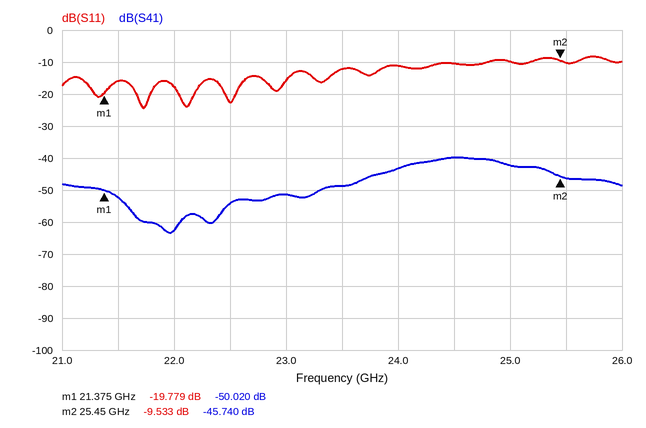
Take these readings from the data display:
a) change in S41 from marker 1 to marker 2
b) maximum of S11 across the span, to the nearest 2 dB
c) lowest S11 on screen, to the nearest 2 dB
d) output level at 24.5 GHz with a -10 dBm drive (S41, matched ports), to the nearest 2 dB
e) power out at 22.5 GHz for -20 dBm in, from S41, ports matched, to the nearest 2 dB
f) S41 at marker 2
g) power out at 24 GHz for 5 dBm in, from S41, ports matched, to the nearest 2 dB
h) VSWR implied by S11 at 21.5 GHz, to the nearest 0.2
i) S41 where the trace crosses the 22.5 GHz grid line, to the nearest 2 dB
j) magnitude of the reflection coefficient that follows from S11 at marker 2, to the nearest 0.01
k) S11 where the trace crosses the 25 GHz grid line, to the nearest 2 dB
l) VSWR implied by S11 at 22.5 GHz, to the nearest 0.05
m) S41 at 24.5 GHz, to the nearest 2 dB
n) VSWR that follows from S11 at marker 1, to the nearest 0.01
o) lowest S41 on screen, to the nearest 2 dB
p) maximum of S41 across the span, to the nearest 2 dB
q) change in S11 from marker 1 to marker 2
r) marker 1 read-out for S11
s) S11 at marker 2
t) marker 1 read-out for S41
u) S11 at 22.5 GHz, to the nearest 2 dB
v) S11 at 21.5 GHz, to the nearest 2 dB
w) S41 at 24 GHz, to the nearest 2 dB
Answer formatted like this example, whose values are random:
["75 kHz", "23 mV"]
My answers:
["4.280 dB", "-8 dB", "-24 dB", "-50 dBm", "-74 dBm", "-45.740 dB", "-38 dBm", "1.4", "-54 dB", "0.33", "-10 dB", "1.15", "-40 dB", "1.23", "-64 dB", "-40 dB", "10.246 dB", "-19.779 dB", "-9.533 dB", "-50.020 dB", "-22 dB", "-16 dB", "-44 dB"]
